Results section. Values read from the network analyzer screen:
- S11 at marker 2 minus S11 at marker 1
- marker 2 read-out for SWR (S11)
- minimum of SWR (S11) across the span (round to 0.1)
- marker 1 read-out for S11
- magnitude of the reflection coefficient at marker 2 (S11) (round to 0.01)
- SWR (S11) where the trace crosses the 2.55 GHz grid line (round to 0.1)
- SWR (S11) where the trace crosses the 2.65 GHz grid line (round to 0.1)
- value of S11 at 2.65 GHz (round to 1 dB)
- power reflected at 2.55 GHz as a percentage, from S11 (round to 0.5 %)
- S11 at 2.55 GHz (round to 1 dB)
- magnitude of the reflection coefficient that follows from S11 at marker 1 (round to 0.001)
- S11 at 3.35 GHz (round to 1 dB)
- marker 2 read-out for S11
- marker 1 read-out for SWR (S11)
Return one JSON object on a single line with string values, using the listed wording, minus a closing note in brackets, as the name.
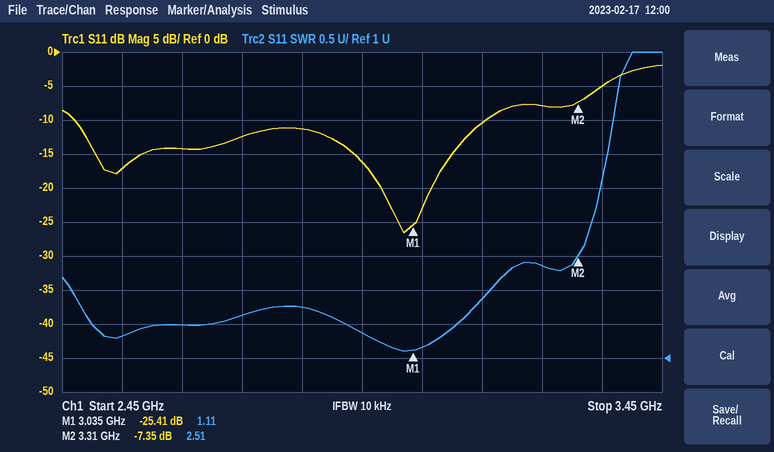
{"S11 at marker 2 minus S11 at marker 1": "18.06 dB", "marker 2 read-out for SWR": "2.51", "minimum of SWR (S11) across the span": "1.1", "marker 1 read-out for S11": "-25.41 dB", "magnitude of the reflection coefficient at marker 2 (S11)": "0.43", "SWR (S11) where the trace crosses the 2.55 GHz grid line": "1.3", "SWR (S11) where the trace crosses the 2.65 GHz grid line": "1.5", "value of S11 at 2.65 GHz": "-14 dB", "power reflected at 2.55 GHz as a percentage, from S11": "2.0 %", "S11 at 2.55 GHz": "-17 dB", "magnitude of the reflection coefficient that follows from S11 at marker 1": "0.054", "S11 at 3.35 GHz": "-5 dB", "marker 2 read-out for S11": "-7.35 dB", "marker 1 read-out for SWR": "1.11"}
